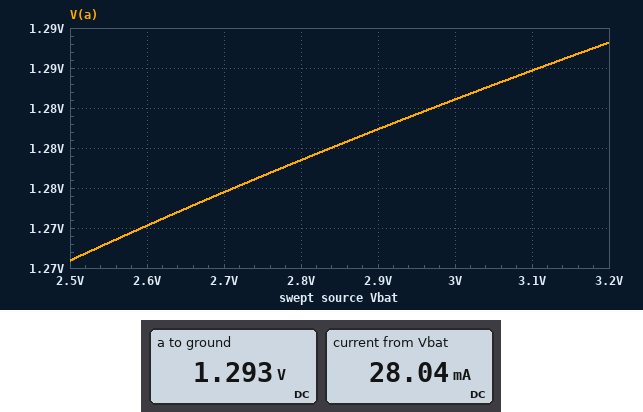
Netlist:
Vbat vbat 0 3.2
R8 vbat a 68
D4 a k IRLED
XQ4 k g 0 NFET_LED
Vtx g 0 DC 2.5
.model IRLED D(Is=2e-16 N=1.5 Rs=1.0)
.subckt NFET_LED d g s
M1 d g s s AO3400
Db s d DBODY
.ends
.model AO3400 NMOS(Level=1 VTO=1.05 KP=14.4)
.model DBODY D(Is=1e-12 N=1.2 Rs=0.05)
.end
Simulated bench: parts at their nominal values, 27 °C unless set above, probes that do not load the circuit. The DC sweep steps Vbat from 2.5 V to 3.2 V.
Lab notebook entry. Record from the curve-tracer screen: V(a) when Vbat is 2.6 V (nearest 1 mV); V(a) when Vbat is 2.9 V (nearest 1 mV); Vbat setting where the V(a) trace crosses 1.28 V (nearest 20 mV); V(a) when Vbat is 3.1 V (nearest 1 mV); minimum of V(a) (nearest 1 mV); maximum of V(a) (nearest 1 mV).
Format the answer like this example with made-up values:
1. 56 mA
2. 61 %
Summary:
1. 1.270 V
2. 1.282 V
3. 2.84 V
4. 1.290 V
5. 1.266 V
6. 1.293 V
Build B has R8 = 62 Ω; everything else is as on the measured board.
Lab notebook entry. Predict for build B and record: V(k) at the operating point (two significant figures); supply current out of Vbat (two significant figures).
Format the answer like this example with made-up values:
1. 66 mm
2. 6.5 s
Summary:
1. 1.5 mV
2. 31 mA
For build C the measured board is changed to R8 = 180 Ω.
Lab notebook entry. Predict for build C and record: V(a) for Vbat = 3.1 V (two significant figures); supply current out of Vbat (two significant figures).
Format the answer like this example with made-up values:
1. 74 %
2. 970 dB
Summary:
1. 1.2 V
2. 11 mA
